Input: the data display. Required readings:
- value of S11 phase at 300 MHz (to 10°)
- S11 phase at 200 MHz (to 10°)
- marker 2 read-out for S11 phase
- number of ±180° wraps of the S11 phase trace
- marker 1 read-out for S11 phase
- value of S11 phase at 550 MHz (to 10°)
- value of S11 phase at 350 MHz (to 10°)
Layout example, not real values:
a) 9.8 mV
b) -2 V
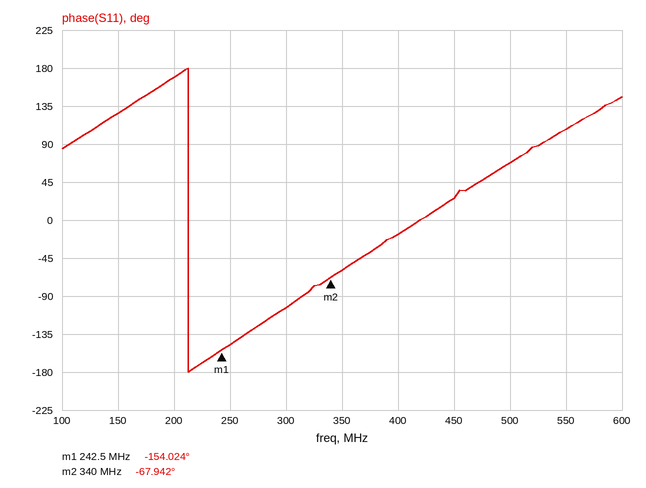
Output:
a) -100°
b) 170°
c) -67.942°
d) 1
e) -154.024°
f) 110°
g) -60°
